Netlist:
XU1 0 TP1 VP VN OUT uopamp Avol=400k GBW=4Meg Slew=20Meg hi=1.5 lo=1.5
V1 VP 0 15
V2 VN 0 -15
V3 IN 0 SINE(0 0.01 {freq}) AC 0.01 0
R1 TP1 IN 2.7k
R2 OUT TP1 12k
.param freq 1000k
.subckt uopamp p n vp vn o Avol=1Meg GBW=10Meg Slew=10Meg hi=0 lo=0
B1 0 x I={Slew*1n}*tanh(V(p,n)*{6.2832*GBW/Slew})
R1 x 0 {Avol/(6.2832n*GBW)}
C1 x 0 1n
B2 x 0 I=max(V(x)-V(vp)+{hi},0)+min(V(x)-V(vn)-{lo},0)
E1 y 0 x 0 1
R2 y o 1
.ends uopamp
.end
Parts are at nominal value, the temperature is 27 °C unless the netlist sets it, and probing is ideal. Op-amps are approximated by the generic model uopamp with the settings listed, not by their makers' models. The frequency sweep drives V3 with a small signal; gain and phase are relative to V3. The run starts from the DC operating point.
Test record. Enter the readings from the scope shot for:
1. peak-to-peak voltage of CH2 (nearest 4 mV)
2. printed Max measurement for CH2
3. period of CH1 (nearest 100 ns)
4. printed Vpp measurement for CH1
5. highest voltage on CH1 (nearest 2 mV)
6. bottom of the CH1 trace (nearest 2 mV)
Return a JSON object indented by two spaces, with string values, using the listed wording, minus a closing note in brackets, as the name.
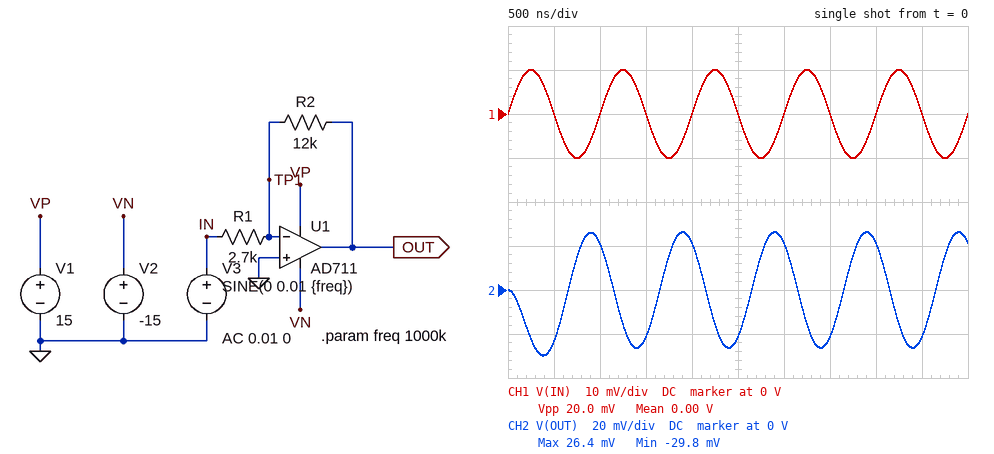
{
  "peak-to-peak voltage of CH2": "56 mV",
  "printed Max measurement for CH2": "26.4 mV",
  "period of CH1": "1.0 µs",
  "printed Vpp measurement for CH1": "20.0 mV",
  "highest voltage on CH1": "10 mV",
  "bottom of the CH1 trace": "-10 mV"
}
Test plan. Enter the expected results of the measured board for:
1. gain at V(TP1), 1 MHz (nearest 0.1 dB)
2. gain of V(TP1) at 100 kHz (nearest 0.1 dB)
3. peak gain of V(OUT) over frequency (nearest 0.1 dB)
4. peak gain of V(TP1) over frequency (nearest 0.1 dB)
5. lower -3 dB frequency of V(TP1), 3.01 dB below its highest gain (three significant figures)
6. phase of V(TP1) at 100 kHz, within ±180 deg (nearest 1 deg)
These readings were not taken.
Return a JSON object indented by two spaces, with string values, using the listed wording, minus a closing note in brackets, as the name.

{
  "gain at V(TP1), 1 MHz": "-3.6 dB",
  "gain of V(TP1) at 100 kHz": "-19.2 dB",
  "peak gain of V(OUT) over frequency": "13.0 dB",
  "peak gain of V(TP1) over frequency": "-1.8 dB",
  "lower -3 dB frequency of V(TP1), 3.01 dB below its highest gain": "735 kHz",
  "phase of V(TP1) at 100 kHz, within ±180 deg": "82 deg"
}
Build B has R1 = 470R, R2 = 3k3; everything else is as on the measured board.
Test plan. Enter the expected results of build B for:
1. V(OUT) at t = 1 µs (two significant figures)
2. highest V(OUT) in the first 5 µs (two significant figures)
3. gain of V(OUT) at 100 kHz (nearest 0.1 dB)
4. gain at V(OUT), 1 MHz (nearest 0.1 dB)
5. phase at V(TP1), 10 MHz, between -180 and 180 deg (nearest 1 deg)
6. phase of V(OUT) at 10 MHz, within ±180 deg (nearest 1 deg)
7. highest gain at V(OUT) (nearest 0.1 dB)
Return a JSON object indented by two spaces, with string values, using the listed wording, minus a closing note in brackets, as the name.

{
  "V(OUT) at t = 1 µs": "27 mV",
  "highest V(OUT) in the first 5 µs": "31 mV",
  "gain of V(OUT) at 100 kHz": "16.8 dB",
  "gain at V(OUT), 1 MHz": "9.9 dB",
  "phase at V(TP1), 10 MHz, between -180 and 180 deg": "3 deg",
  "phase of V(OUT) at 10 MHz, within ±180 deg": "93 deg",
  "highest gain at V(OUT)": "16.9 dB"
}
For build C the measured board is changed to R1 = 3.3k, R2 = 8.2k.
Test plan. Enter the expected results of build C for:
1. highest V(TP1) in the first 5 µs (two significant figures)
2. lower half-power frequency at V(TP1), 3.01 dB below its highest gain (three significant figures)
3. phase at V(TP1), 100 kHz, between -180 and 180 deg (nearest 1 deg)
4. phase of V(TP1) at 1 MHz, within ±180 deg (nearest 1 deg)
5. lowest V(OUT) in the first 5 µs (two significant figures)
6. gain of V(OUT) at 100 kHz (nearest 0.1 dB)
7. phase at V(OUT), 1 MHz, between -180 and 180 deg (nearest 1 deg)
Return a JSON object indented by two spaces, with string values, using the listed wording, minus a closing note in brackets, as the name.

{
  "highest V(TP1) in the first 5 µs": "4.7 mV",
  "lower half-power frequency at V(TP1), 3.01 dB below its highest gain": "1.15 MHz",
  "phase at V(TP1), 100 kHz, between -180 and 180 deg": "85 deg",
  "phase of V(TP1) at 1 MHz, within ±180 deg": "49 deg",
  "lowest V(OUT) in the first 5 µs": "-20 mV",
  "gain of V(OUT) at 100 kHz": "7.9 dB",
  "phase at V(OUT), 1 MHz, between -180 and 180 deg": "139 deg"
}
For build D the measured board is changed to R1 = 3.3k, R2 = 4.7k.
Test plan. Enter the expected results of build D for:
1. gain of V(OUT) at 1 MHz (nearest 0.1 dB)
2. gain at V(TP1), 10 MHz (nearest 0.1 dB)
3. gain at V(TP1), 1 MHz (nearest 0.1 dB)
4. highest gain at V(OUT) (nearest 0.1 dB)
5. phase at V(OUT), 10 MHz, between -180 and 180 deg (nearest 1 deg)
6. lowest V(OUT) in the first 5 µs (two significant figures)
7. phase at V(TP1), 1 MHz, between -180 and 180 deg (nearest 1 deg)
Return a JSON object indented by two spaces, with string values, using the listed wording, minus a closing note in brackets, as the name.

{
  "gain of V(OUT) at 1 MHz": "1.7 dB",
  "gain at V(TP1), 10 MHz": "-4.7 dB",
  "gain at V(TP1), 1 MHz": "-10.3 dB",
  "highest gain at V(OUT)": "3.1 dB",
  "phase at V(OUT), 10 MHz, between -180 and 180 deg": "99 deg",
  "lowest V(OUT) in the first 5 µs": "-12 mV",
  "phase at V(TP1), 1 MHz, between -180 and 180 deg": "59 deg"
}
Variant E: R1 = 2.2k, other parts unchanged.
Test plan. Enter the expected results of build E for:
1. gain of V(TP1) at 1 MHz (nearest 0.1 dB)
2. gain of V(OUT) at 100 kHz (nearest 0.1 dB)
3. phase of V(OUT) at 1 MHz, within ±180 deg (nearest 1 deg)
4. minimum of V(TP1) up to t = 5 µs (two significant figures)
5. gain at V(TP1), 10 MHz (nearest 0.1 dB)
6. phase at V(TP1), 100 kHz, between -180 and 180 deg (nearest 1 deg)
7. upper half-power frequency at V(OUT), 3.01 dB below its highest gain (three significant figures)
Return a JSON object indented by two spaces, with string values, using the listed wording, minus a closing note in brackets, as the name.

{
  "gain of V(TP1) at 1 MHz": "-2.9 dB",
  "gain of V(OUT) at 100 kHz": "14.6 dB",
  "phase of V(OUT) at 1 MHz, within ±180 deg": "122 deg",
  "minimum of V(TP1) up to t = 5 µs": "-7.5 mV",
  "gain at V(TP1), 10 MHz": "-1.5 dB",
  "phase at V(TP1), 100 kHz, between -180 and 180 deg": "81 deg",
  "upper half-power frequency at V(OUT), 3.01 dB below its highest gain": "620 kHz"
}
